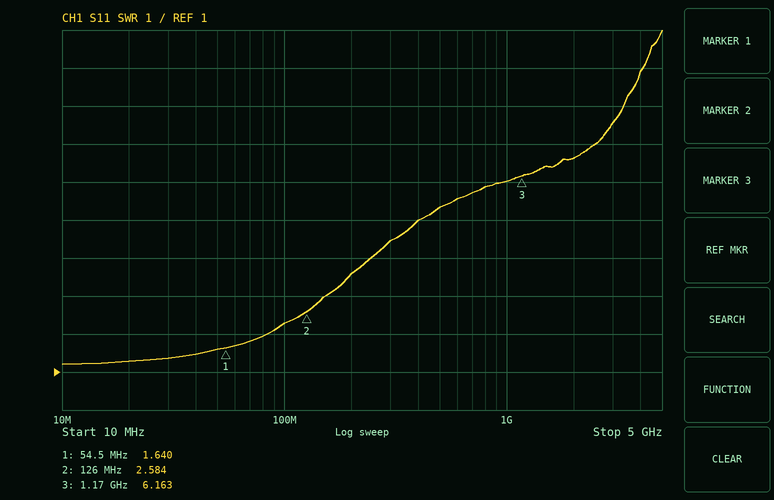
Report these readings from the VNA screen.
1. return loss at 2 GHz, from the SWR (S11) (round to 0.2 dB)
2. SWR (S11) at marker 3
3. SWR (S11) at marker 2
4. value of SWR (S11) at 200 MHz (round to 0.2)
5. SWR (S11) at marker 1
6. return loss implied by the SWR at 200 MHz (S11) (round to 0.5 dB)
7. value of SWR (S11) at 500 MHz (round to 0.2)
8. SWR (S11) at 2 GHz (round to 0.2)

2.6 dB
6.163
2.584
3.6
1.640
5.0 dB
5.4
6.6
